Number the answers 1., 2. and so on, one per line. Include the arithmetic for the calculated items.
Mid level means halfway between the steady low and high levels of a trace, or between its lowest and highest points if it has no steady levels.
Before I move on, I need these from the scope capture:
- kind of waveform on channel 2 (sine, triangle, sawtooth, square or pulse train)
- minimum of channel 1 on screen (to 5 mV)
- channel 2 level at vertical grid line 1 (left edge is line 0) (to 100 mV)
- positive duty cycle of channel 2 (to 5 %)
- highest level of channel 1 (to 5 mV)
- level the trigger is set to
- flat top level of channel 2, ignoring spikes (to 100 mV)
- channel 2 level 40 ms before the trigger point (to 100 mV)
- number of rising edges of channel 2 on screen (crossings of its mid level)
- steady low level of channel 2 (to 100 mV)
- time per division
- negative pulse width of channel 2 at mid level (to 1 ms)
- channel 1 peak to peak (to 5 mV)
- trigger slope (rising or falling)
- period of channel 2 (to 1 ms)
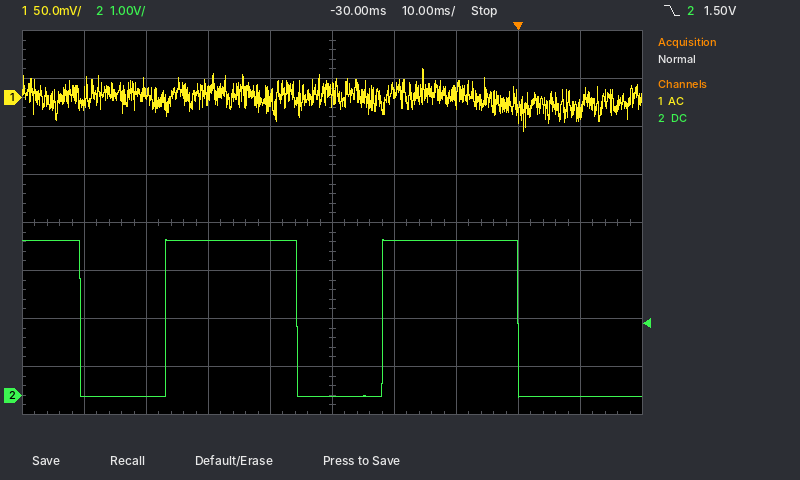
1. pulse train
2. -35 mV
3. 0.0 V
4. 60 %
5. 30 mV
6. 1.50 V
7. 3.2 V
8. 3.2 V
9. 2
10. 0.0 V
11. 10 ms
12. 14 ms
13. 30 mV − (-35 mV) = 65 mV
14. falling
15. 35 ms
